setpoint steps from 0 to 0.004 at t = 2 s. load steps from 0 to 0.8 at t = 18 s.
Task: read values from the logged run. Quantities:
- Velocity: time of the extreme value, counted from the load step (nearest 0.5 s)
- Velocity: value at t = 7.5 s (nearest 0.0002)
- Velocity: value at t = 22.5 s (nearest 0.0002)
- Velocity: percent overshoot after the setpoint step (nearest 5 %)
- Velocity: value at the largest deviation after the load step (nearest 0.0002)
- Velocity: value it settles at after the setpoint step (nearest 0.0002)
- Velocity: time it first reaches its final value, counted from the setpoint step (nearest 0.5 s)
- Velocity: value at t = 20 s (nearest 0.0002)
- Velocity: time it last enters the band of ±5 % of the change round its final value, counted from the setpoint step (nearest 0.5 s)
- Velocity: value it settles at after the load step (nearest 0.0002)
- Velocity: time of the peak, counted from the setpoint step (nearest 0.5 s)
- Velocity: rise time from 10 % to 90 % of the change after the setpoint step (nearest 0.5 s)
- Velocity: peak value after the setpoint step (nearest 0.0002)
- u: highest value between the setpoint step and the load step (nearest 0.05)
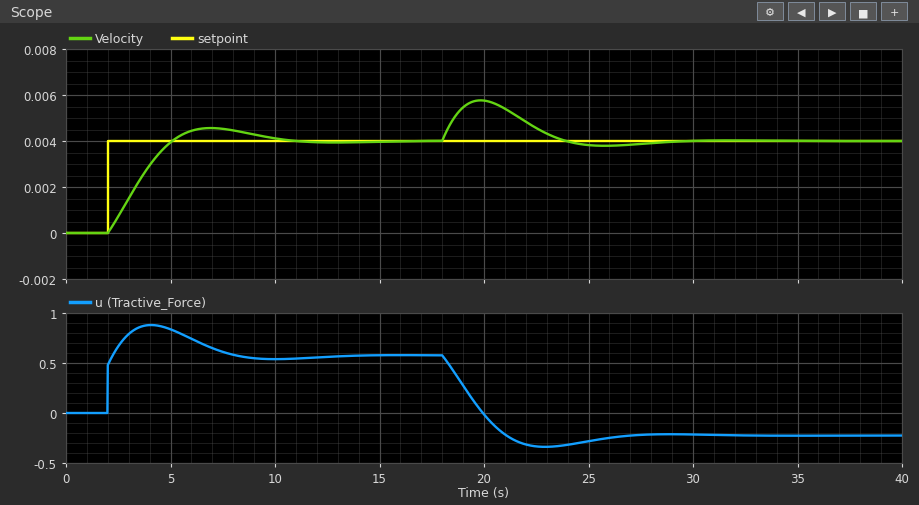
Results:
2.0 s
0.0046
0.0046
15 %
0.0058
0.0040
3.0 s
0.0058
7.5 s
0.0040
5.0 s
2.5 s
0.0046
0.90
